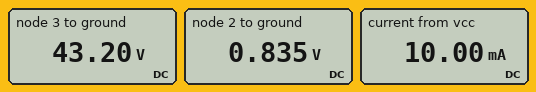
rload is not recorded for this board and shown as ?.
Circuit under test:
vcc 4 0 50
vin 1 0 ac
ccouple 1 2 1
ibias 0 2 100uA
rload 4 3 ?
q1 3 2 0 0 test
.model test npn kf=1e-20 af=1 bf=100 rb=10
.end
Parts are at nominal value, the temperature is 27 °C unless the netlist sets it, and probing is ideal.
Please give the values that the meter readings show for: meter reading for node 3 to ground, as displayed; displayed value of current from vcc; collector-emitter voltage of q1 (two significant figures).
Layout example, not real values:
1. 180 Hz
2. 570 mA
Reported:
1. 43.20 V
2. 10.00 mA
3. 43 V
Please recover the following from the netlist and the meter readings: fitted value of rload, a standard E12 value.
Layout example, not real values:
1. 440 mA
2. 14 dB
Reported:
1. 680 Ω
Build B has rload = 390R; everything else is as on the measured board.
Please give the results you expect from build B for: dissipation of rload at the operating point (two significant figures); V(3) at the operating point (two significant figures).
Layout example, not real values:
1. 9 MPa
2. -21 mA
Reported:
1. 39 mW
2. 46 V
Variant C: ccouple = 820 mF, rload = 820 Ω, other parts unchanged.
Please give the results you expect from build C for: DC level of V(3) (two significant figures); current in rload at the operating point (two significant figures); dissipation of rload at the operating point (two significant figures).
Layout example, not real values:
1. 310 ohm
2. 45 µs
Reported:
1. 42 V
2. 10 mA
3. 82 mW
